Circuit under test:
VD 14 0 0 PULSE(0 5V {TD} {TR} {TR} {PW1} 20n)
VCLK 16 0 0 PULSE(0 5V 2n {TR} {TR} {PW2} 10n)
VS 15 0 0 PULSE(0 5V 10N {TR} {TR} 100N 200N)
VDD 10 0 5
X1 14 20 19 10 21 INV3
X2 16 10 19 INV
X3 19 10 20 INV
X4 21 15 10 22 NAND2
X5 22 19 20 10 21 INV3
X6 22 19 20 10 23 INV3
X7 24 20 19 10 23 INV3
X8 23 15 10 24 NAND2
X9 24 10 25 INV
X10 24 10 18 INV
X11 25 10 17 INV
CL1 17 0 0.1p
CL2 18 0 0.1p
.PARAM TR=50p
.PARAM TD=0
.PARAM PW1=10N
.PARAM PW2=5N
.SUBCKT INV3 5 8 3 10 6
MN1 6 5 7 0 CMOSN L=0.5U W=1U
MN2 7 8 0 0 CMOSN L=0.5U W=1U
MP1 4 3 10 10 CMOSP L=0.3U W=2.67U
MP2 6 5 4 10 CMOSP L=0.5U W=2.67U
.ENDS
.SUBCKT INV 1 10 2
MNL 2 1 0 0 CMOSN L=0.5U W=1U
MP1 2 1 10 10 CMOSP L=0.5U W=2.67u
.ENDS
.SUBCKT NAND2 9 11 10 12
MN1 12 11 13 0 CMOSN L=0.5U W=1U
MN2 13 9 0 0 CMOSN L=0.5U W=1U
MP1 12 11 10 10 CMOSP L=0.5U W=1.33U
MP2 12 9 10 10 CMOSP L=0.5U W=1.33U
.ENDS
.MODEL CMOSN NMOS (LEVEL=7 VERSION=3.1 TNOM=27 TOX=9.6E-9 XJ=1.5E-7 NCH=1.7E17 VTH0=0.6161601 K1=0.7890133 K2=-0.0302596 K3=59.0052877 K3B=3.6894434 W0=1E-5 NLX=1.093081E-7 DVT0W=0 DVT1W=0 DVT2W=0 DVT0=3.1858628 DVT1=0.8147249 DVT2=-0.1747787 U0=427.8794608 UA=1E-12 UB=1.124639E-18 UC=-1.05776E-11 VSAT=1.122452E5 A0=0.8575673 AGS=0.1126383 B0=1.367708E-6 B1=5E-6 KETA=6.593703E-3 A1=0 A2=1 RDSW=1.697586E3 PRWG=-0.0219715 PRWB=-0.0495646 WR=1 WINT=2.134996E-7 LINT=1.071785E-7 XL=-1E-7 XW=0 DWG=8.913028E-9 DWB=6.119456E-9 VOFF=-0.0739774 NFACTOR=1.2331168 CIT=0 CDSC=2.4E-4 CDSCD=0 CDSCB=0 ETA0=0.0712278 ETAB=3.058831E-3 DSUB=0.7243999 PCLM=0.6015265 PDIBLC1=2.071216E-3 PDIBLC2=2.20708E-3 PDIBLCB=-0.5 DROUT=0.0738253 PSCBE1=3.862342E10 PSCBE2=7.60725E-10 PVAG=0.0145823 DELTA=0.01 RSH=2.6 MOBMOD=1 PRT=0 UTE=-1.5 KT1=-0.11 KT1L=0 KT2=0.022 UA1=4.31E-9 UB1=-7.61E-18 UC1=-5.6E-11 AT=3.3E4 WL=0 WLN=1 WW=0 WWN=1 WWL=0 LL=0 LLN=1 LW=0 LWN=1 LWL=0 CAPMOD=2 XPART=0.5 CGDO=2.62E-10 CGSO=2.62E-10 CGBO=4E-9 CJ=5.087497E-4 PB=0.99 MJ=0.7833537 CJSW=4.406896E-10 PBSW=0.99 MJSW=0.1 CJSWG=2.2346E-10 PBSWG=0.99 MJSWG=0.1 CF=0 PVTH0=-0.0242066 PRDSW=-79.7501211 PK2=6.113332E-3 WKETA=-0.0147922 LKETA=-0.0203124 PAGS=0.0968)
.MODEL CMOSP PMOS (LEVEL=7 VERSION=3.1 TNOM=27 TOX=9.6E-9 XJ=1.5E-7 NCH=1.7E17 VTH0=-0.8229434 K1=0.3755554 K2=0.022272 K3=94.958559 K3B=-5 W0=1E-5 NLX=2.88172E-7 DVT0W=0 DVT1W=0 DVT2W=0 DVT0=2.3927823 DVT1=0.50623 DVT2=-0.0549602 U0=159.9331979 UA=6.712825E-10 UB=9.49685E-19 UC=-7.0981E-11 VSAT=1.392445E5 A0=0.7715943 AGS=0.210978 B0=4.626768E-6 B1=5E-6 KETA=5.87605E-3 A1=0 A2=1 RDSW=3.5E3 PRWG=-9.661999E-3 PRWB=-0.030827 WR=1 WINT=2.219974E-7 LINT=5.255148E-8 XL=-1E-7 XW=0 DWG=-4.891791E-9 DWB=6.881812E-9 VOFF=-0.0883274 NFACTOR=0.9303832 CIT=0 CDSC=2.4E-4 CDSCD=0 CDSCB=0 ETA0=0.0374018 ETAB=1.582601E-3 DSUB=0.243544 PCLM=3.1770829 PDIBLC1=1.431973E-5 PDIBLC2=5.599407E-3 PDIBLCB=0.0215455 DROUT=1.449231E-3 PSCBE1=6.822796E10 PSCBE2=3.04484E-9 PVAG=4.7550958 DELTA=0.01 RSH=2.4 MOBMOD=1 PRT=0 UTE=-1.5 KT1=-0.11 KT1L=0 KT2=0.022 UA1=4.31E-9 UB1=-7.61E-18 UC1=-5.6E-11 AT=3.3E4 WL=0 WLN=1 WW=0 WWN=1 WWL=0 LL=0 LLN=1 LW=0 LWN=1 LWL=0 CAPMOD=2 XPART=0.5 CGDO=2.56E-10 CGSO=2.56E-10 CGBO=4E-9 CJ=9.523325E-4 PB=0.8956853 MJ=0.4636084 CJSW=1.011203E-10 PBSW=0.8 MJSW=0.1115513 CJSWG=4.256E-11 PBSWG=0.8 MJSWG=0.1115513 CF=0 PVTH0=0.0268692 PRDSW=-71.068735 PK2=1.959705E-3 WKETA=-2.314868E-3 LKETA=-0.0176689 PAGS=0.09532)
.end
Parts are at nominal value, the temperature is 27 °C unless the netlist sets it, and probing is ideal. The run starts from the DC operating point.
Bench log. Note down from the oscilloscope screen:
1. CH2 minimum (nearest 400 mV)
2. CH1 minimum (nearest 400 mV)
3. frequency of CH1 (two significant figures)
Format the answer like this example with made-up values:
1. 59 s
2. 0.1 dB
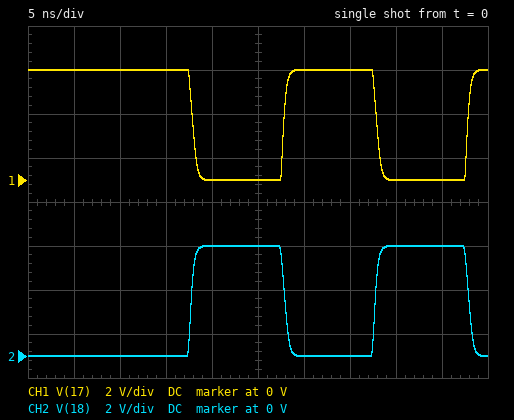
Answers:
1. 0 V
2. 0 V
3. 50 MHz
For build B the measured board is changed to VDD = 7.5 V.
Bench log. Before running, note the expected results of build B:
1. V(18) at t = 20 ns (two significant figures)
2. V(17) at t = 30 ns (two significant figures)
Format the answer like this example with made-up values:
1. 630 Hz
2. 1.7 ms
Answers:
1. 7.4 V
2. 7.5 V
